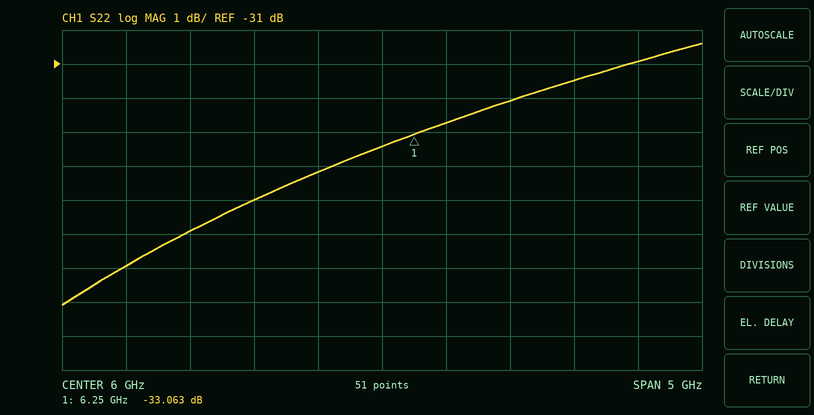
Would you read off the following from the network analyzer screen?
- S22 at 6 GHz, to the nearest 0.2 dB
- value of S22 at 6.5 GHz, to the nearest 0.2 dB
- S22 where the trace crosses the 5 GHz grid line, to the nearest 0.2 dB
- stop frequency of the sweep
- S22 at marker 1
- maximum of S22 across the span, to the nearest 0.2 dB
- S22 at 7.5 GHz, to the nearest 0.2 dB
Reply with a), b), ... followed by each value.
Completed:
a) -33.4 dB
b) -32.8 dB
c) -35.0 dB
d) 8.5 GHz
e) -33.063 dB
f) -30.4 dB
g) -31.4 dB
